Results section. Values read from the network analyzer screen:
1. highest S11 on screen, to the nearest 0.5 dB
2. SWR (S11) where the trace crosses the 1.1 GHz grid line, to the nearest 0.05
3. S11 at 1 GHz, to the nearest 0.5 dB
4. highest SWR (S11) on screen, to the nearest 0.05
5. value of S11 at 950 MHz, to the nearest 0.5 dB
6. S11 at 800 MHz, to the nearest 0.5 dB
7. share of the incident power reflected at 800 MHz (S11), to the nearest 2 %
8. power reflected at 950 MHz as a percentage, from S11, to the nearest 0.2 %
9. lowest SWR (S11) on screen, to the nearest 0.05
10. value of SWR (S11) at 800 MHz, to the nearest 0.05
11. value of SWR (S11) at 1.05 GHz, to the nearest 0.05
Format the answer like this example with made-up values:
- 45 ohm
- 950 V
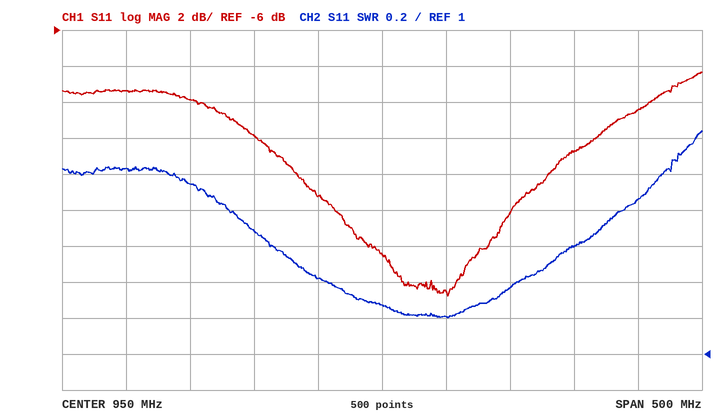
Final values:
- -8.5 dB
- 1.60
- -20.5 dB
- 2.25
- -18.5 dB
- -10.0 dB
- 10 %
- 1.4 %
- 1.20
- 1.95
- 1.35
